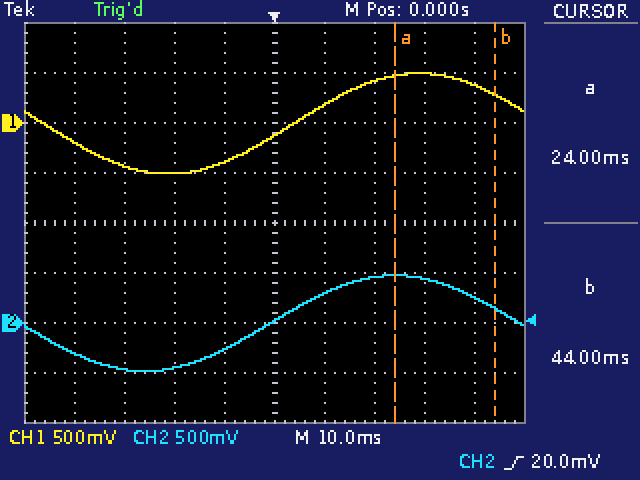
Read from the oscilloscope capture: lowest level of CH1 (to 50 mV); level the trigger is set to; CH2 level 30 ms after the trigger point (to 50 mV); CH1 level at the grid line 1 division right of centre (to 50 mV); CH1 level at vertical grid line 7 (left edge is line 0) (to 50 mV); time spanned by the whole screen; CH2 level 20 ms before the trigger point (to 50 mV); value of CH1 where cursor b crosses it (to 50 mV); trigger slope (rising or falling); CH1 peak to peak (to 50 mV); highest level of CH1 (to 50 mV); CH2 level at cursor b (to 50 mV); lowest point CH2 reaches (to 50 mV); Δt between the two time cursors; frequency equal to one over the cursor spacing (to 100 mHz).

-500 mV
20.0 mV
450 mV
200 mV
400 mV
100 ms
-450 mV
300 mV
rising
1.00 V
500 mV
150 mV
-500 mV
20 ms
50.0 Hz
